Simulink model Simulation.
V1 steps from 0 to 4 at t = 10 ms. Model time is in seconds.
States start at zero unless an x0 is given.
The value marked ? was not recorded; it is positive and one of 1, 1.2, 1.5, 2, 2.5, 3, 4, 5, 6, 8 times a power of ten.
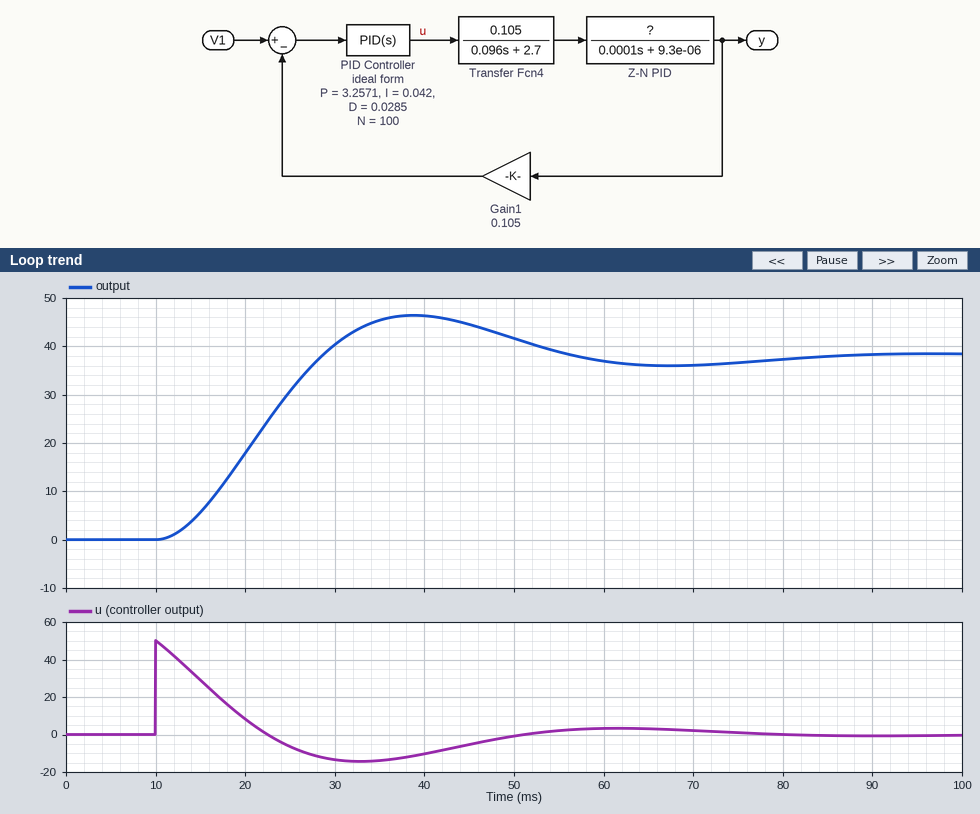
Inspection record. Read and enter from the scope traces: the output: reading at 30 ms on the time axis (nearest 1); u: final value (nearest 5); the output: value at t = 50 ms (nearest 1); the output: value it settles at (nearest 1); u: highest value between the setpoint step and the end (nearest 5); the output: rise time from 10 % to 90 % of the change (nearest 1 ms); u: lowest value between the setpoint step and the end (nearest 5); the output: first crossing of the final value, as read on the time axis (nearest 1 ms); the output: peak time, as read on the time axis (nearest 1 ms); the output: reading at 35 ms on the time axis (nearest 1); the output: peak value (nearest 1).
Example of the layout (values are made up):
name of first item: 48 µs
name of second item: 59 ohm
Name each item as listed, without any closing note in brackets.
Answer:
the output: reading at 30 ms on the time axis: 40
u: final value: 0
the output: value at t = 50 ms: 42
the output: value it settles at: 38
u: highest value between the setpoint step and the end: 50
the output: rise time from 10 % to 90 % of the change: 13 ms
u: lowest value between the setpoint step and the end: -15
the output: first crossing of the final value, as read on the time axis: 29 ms
the output: peak time, as read on the time axis: 39 ms
the output: reading at 35 ms on the time axis: 45
the output: peak value: 46
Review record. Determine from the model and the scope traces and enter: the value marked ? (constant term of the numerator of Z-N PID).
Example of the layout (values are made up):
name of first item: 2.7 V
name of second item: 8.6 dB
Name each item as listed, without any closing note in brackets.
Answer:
the value marked ?: 1
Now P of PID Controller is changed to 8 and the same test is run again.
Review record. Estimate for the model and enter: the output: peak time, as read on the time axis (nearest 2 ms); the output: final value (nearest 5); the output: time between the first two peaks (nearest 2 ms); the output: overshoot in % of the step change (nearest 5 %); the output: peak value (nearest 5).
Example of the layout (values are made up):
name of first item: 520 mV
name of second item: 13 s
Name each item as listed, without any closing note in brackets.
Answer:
the output: peak time, as read on the time axis: 28 ms
the output: final value: 40
the output: time between the first two peaks: 34 ms
the output: overshoot in % of the step change: 40 %
the output: peak value: 55
